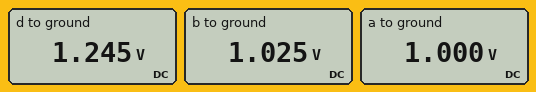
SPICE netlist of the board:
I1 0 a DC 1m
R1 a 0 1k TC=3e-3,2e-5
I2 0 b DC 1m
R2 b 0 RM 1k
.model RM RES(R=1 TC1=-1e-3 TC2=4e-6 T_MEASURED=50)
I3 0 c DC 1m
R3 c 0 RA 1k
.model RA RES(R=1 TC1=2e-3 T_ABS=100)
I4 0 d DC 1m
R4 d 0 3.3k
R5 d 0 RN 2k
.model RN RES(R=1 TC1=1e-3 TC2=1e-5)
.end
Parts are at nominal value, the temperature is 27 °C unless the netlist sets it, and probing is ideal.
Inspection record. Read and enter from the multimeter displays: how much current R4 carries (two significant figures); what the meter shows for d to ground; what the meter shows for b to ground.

380 µA
1.245 V
1.025 V
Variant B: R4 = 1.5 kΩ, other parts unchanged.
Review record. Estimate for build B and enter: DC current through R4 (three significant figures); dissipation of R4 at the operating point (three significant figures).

571 µA
490 µW
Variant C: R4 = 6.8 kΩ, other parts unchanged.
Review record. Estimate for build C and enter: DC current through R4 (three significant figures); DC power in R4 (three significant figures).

227 µA
351 µW
